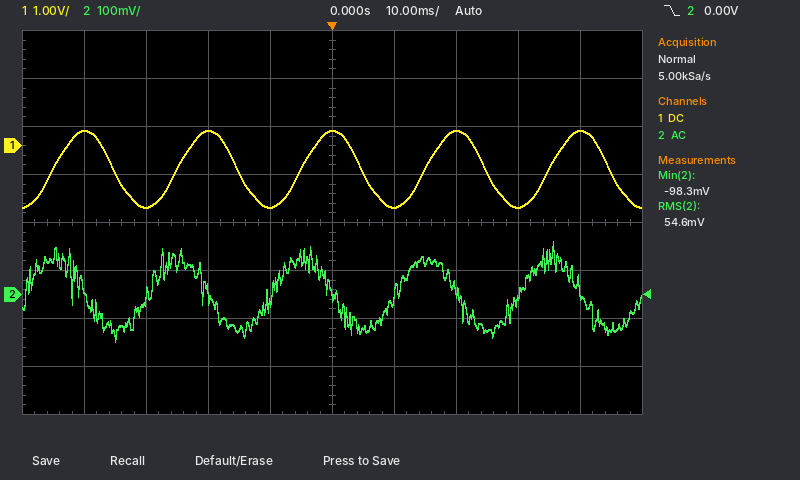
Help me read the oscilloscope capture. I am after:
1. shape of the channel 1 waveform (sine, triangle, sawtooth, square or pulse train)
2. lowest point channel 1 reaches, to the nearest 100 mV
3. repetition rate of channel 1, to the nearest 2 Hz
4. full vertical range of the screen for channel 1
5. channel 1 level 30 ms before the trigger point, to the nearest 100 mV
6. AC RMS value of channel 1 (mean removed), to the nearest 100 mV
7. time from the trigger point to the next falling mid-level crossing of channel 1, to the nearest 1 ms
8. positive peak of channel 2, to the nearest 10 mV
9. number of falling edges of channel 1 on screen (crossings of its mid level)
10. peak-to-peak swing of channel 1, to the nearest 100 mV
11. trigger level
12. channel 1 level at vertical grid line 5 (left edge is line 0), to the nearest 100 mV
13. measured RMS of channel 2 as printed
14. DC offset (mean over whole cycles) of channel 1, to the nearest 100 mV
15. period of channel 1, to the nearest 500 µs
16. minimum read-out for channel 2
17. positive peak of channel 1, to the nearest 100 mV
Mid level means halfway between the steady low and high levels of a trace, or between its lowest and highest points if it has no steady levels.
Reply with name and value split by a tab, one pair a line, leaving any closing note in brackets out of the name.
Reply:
shape of the channel 1 waveform	sine
lowest point channel 1 reaches, to the nearest 100 mV	-1.3 V
repetition rate of channel 1, to the nearest 2 Hz	50 Hz
full vertical range of the screen for channel 1	8 V
channel 1 level 30 ms before the trigger point, to the nearest 100 mV	-1.3 V
AC RMS value of channel 1 (mean removed), to the nearest 100 mV	600 mV
time from the trigger point to the next falling mid-level crossing of channel 1, to the nearest 1 ms	5 ms
positive peak of channel 2, to the nearest 10 mV	110 mV
number of falling edges of channel 1 on screen	5
peak-to-peak swing of channel 1, to the nearest 100 mV	1.6 V
trigger level	0.00 V
channel 1 level at vertical grid line 5 (left edge is line 0), to the nearest 100 mV	300 mV
measured RMS of channel 2 as printed	54.6 mV
DC offset (mean over whole cycles) of channel 1, to the nearest 100 mV	-500 mV
period of channel 1, to the nearest 500 µs	20.0 ms
minimum read-out for channel 2	-98.3 mV
positive peak of channel 1, to the nearest 100 mV	300 mV
